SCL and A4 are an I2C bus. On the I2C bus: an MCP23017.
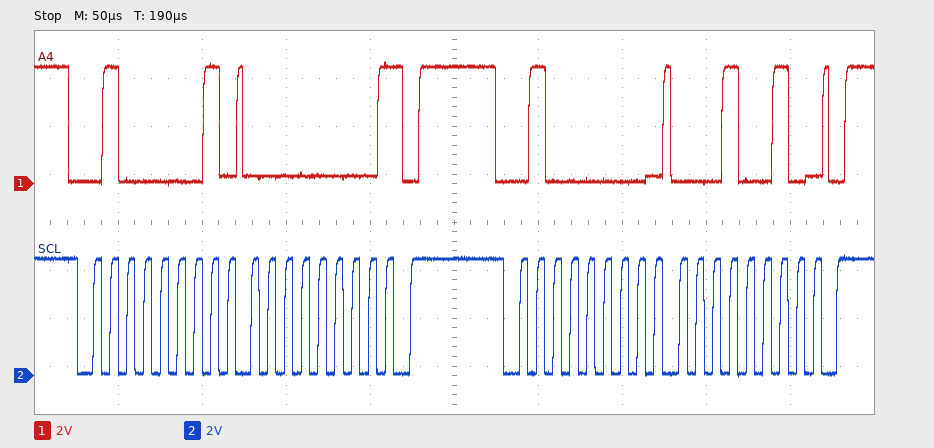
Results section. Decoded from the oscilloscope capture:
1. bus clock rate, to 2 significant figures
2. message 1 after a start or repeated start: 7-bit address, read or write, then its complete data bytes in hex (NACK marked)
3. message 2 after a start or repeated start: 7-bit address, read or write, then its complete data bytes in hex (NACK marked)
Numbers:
100 kHz
0x20 read: 00 NACK
0x20 write: 12
